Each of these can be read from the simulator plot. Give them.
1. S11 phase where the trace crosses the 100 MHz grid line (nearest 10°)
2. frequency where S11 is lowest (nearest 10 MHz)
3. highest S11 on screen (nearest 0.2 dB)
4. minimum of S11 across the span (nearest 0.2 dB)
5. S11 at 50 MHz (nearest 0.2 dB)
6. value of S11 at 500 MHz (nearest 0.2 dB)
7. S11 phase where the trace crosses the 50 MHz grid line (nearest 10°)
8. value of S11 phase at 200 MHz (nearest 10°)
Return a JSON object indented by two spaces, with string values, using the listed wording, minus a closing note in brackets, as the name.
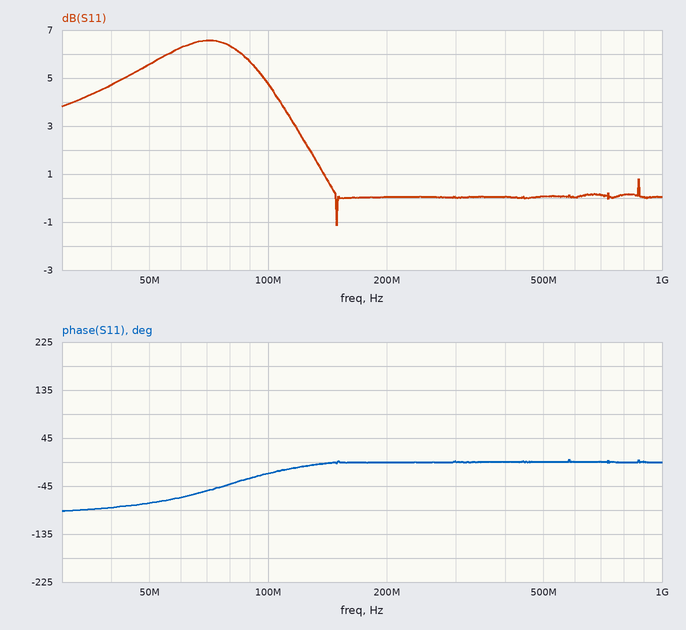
{
  "S11 phase where the trace crosses the 100 MHz grid line": "-20°",
  "frequency where S11 is lowest": "150 MHz",
  "highest S11 on screen": "6.6 dB",
  "minimum of S11 across the span": "-1.2 dB",
  "S11 at 50 MHz": "5.6 dB",
  "value of S11 at 500 MHz": "0.0 dB",
  "S11 phase where the trace crosses the 50 MHz grid line": "-80°",
  "value of S11 phase at 200 MHz": "0°"
}
